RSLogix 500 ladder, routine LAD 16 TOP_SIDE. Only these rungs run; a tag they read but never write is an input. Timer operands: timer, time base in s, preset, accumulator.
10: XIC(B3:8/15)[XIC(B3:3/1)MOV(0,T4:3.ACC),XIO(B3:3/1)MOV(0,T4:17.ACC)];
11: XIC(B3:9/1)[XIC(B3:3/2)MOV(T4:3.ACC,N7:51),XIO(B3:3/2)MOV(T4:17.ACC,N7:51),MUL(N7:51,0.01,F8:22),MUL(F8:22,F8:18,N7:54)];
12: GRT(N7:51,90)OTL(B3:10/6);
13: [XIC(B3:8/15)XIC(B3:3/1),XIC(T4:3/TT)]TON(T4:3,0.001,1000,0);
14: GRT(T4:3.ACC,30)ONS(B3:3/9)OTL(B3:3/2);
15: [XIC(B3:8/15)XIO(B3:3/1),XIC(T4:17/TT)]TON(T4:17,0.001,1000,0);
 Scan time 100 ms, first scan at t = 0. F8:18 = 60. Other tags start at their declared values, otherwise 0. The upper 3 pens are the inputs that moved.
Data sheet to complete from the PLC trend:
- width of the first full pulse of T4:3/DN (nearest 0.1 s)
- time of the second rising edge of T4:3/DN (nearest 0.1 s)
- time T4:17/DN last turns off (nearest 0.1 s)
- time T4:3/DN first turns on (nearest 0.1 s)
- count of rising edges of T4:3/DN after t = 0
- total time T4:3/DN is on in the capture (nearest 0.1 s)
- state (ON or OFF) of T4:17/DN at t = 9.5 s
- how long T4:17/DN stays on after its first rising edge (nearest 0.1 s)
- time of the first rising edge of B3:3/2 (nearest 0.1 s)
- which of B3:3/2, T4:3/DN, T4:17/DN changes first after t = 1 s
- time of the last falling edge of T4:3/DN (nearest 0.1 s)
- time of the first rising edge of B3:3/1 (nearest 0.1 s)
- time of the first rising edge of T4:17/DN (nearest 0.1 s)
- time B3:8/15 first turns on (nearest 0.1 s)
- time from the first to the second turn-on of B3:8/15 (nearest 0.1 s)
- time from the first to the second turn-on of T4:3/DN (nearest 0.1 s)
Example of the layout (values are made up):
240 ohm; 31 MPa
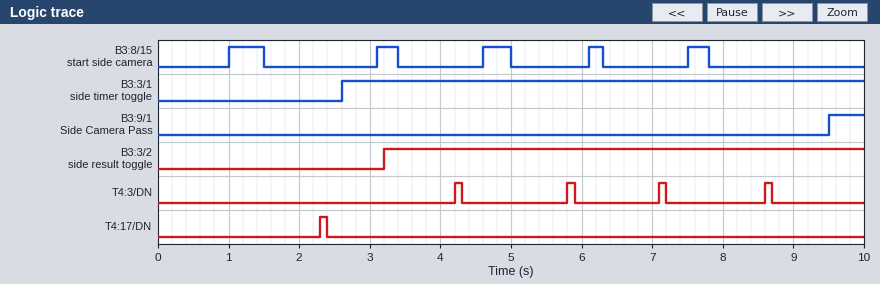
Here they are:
0.1 s; 5.8 s; 2.4 s; 4.2 s; 4; 0.4 s; OFF; 0.1 s; 3.2 s; T4:17/DN; 8.7 s; 2.6 s; 2.3 s; 1.0 s; 2.1 s; 1.6 s
